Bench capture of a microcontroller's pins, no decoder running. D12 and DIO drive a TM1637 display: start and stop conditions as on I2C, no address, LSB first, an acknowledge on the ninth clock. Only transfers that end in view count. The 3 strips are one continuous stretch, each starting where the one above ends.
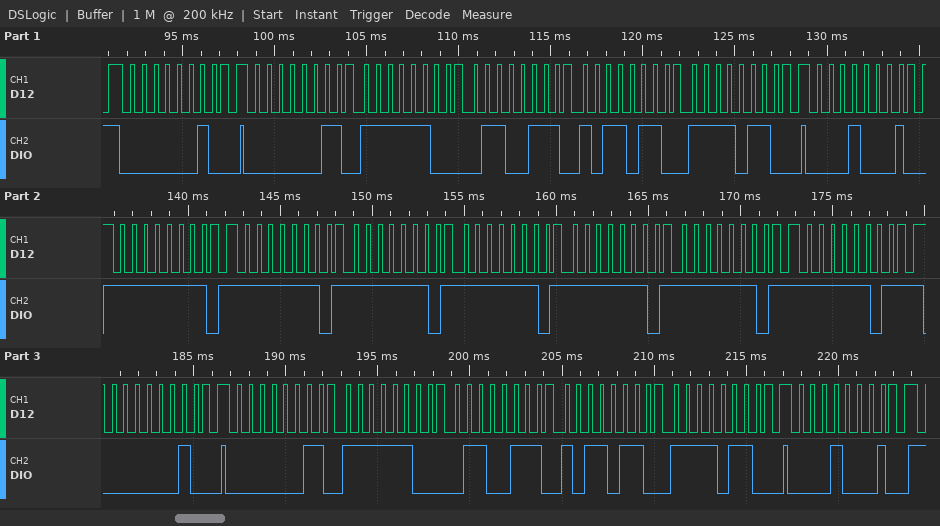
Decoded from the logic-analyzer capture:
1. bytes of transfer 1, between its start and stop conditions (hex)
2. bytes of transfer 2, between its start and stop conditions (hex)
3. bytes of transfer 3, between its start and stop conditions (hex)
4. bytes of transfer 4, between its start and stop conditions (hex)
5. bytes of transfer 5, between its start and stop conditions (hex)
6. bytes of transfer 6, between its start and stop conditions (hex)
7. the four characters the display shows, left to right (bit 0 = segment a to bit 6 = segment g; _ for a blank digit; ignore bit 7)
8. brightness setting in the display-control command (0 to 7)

40
C0 3F E6 6D 6F
88
40
C0 3F E6 6D 6F
88
0459
0
